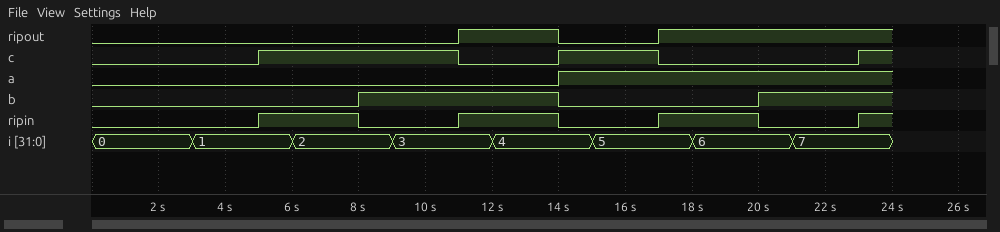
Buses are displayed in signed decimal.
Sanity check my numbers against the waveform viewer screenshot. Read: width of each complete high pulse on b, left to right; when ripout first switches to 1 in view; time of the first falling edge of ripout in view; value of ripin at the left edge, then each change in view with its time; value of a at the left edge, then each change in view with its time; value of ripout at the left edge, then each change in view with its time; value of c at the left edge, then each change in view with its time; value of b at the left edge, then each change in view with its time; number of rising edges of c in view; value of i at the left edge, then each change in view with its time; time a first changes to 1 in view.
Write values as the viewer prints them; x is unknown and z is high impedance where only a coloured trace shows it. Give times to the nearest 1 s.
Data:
6 s
11 s
14 s
0, 1 at 5 s, 0 at 8 s, 1 at 11 s, 0 at 14 s, 1 at 17 s, 0 at 20 s, 1 at 23 s
0, 1 at 14 s
0, 1 at 11 s, 0 at 14 s, 1 at 17 s
0, 1 at 5 s, 0 at 11 s, 1 at 14 s, 0 at 17 s, 1 at 23 s
0, 1 at 8 s, 0 at 14 s, 1 at 20 s
3
0, 1 at 3 s, 2 at 6 s, 3 at 9 s, 4 at 12 s, 5 at 15 s, 6 at 18 s, 7 at 21 s
14 s
